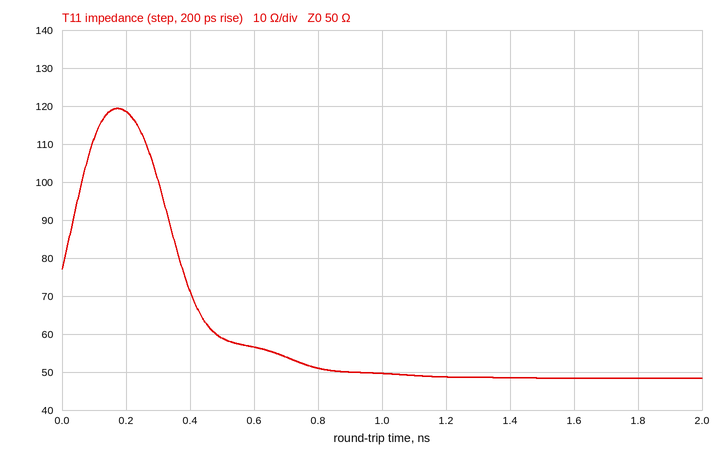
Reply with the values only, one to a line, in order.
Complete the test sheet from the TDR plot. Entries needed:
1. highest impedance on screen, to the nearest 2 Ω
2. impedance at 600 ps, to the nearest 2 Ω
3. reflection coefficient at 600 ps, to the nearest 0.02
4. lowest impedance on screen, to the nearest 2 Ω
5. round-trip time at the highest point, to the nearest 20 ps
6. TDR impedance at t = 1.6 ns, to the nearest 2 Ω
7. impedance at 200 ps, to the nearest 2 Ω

120 Ω
56 Ω
+0.06
48 Ω
180 ps
48 Ω
118 Ω
